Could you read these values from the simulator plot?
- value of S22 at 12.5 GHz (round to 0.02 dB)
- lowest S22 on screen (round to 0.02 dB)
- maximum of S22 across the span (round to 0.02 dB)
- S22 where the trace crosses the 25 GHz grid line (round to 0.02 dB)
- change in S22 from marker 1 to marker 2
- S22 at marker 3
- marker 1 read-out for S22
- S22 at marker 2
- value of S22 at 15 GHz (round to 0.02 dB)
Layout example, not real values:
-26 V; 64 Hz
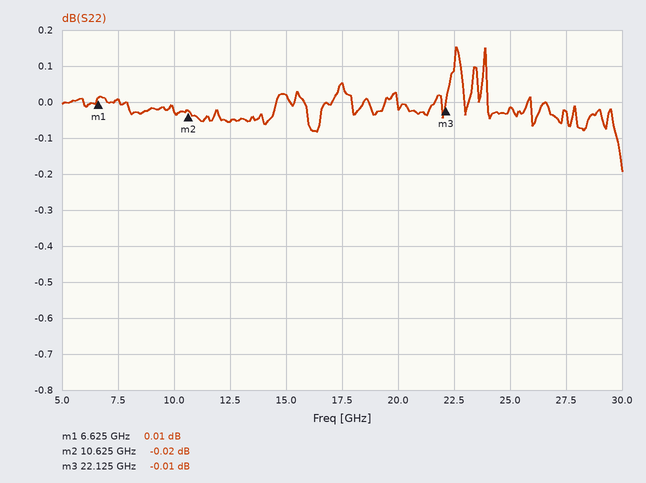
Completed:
-0.06 dB; -0.20 dB; 0.16 dB; -0.02 dB; -0.03 dB; -0.01 dB; 0.01 dB; -0.02 dB; 0.02 dB
